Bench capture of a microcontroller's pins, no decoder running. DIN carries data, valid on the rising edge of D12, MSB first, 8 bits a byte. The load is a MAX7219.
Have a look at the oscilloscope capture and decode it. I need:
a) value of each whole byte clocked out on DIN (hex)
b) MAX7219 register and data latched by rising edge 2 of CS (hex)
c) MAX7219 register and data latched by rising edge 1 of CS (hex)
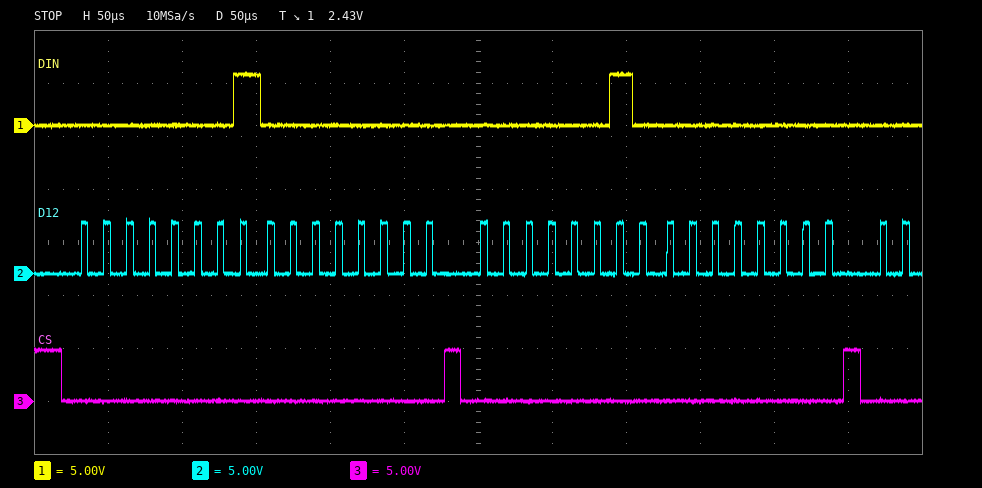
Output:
01 00 02 00
register 0x2, data 0x00
register 0x1, data 0x00
